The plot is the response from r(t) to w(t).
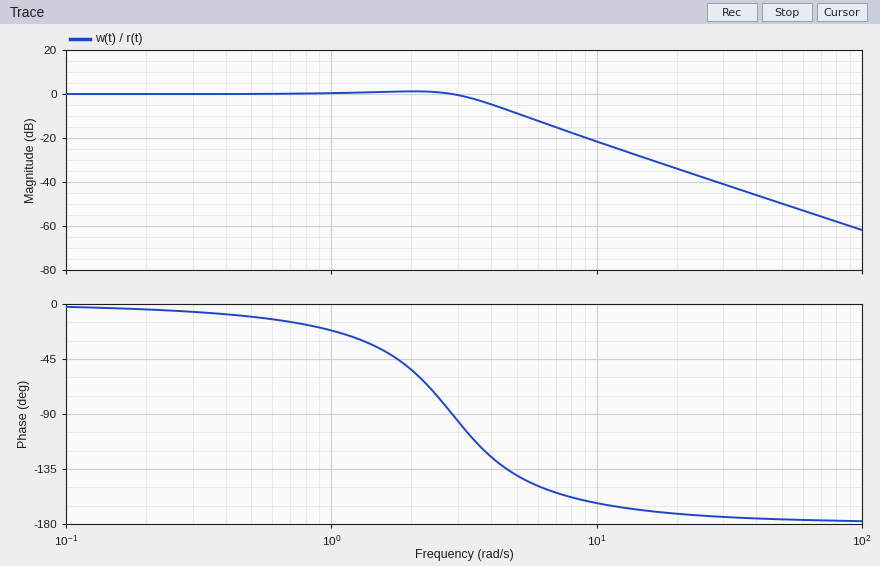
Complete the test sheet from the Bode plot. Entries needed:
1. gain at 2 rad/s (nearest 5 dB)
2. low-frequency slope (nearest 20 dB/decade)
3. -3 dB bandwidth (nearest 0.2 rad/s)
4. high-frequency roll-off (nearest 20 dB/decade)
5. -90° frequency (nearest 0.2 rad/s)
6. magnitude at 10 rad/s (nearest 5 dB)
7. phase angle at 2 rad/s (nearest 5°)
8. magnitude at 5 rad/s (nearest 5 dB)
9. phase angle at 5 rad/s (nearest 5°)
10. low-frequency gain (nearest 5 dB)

0 dB
0 dB/decade
3.6 rad/s
-40 dB/decade
2.8 rad/s
-20 dB
-55°
-10 dB
-140°
0 dB
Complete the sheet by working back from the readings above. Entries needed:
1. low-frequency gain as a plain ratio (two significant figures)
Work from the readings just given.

1.0
